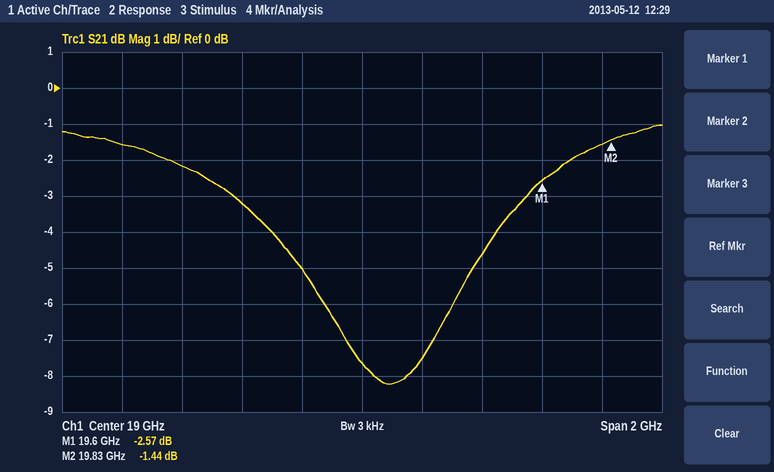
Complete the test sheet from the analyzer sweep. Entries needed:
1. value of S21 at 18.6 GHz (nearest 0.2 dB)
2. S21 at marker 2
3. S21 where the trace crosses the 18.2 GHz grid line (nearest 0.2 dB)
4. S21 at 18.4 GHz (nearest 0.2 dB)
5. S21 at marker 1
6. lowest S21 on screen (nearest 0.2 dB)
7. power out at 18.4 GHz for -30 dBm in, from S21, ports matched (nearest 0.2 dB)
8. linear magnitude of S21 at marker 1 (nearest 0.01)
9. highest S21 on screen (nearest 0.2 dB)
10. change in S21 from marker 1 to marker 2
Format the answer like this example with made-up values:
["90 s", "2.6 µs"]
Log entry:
["-3.2 dB", "-1.44 dB", "-1.6 dB", "-2.2 dB", "-2.57 dB", "-8.2 dB", "-32.2 dBm", "0.74", "-1.0 dB", "1.13 dB"]
